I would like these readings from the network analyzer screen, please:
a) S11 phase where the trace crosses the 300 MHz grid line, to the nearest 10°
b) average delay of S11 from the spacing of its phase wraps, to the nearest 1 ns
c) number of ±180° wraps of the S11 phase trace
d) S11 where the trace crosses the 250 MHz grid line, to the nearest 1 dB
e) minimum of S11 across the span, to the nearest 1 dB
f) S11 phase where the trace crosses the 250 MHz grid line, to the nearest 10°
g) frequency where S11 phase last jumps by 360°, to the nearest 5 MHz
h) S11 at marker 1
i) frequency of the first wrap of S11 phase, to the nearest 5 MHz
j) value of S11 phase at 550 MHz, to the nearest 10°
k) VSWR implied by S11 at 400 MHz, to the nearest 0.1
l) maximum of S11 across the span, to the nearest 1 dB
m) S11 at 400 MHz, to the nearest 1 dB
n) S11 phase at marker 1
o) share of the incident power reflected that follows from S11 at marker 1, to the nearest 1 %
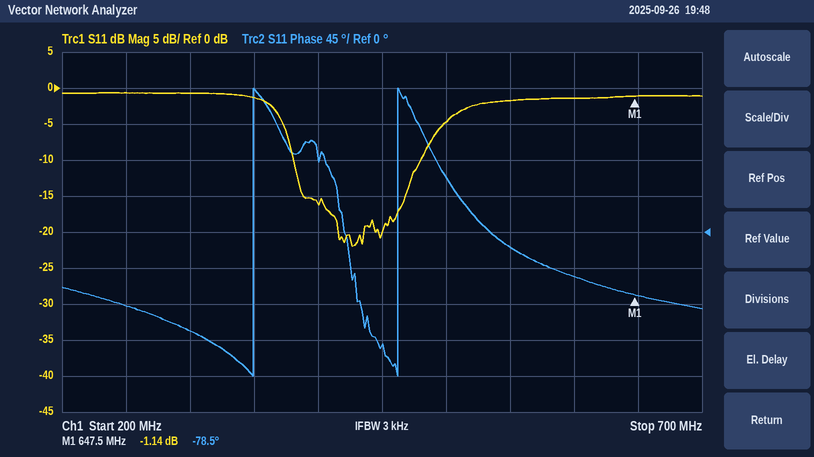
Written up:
-120°
9 ns
2
-1 dB
-22 dB
-90°
460 MHz
-1.14 dB
350 MHz
-20°
1.4
-1 dB
-16 dB
-78.5°
77 %
